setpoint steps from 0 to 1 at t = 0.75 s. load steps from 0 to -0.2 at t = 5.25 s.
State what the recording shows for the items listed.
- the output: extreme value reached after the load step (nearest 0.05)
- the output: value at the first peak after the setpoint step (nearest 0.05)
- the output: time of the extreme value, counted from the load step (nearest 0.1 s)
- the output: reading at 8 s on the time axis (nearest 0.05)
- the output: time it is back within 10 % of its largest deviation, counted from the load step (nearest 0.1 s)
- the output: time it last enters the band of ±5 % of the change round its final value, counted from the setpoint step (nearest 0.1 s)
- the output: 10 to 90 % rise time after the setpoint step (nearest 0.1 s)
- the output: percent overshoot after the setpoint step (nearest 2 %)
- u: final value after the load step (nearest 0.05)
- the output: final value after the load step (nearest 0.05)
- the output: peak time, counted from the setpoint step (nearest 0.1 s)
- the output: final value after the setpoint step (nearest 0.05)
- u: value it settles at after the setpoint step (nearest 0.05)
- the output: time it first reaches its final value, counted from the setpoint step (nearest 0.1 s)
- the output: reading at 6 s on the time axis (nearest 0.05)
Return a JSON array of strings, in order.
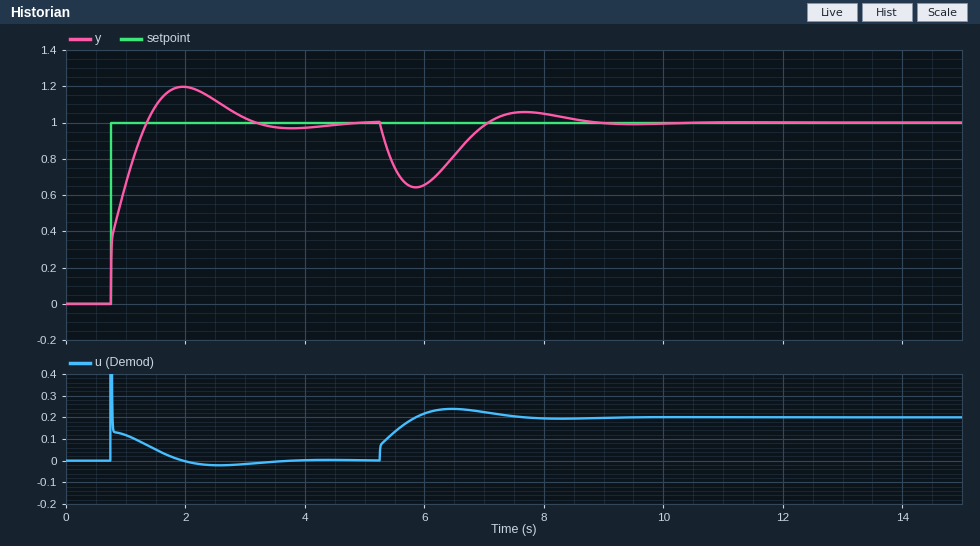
["0.65", "1.20", "0.6 s", "1.05", "3.0 s", "2.1 s", "0.5 s", "20 %", "0.20", "1.00", "1.2 s", "1.00", "0.00", "0.6 s", "0.65"]
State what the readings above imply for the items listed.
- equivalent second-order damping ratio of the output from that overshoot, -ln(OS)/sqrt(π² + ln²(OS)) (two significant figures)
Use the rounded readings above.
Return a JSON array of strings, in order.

["0.46"]
